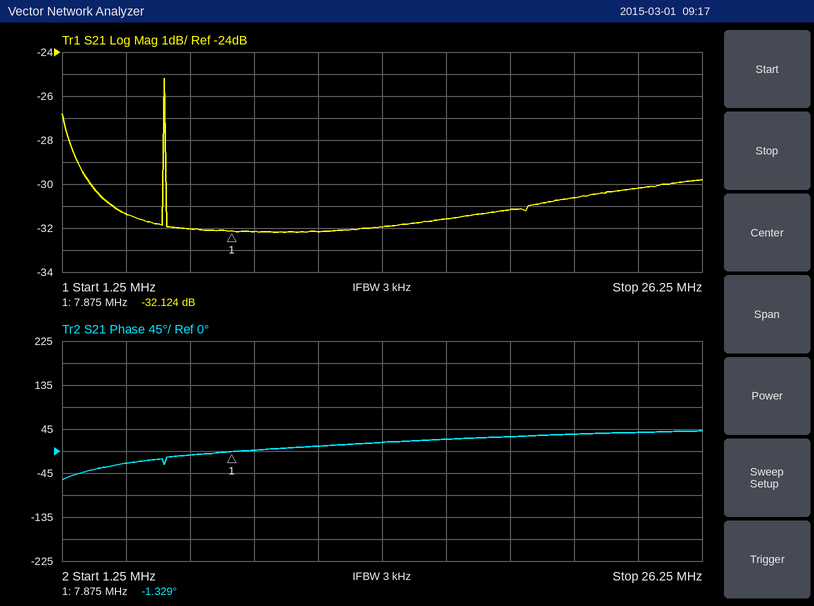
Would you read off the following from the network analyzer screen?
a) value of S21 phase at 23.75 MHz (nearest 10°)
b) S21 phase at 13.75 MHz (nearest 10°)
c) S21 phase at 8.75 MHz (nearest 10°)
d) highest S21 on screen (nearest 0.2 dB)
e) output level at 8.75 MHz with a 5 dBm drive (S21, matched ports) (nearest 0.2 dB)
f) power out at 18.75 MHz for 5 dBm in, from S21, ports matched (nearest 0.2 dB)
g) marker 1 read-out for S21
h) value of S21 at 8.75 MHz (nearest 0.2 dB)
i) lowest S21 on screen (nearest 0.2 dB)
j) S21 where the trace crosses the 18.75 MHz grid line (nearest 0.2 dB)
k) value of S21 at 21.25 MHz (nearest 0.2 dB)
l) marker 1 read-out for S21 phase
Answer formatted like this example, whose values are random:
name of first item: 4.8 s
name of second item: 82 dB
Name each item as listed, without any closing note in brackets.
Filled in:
value of S21 phase at 23.75 MHz: 40°
S21 phase at 13.75 MHz: 20°
S21 phase at 8.75 MHz: 0°
highest S21 on screen: -25.2 dB
output level at 8.75 MHz with a 5 dBm drive (S21, matched ports): -27.2 dBm
power out at 18.75 MHz for 5 dBm in, from S21, ports matched: -26.2 dBm
marker 1 read-out for S21: -32.124 dB
value of S21 at 8.75 MHz: -32.2 dB
lowest S21 on screen: -32.2 dB
S21 where the trace crosses the 18.75 MHz grid line: -31.2 dB
value of S21 at 21.25 MHz: -30.6 dB
marker 1 read-out for S21 phase: -1.329°
